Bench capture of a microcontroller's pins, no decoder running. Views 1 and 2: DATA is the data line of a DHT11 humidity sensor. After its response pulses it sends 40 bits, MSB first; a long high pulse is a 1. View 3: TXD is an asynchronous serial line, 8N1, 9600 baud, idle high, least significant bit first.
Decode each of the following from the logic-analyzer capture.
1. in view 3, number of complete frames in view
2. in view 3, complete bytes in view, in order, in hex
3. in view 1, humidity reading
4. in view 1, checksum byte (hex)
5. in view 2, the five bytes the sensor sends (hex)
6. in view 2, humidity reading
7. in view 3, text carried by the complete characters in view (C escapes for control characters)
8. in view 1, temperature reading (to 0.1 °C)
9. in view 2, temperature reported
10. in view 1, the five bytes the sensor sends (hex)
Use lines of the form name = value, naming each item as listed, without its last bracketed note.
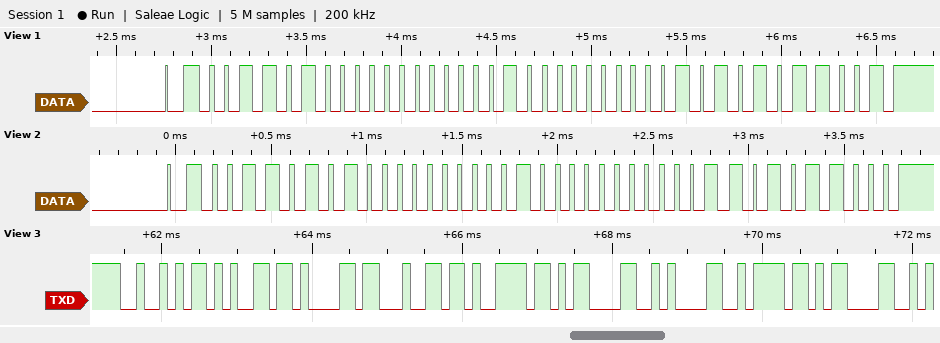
in view 3, number of complete frames in view = 9
in view 3, complete bytes in view, in order, in hex = 0x52 0x65 0x61 0x64 0x79 0x0D 0x0A 0x7A 0x0D
in view 1, humidity reading = 52 %
in view 1, checksum byte = 0x59
in view 2, the five bytes the sensor sends = 35 00 20 03 58
in view 2, humidity reading = 53 %
in view 3, text carried by the complete characters in view = "Ready\r\nz\r"
in view 1, temperature reading = 32.5 °C
in view 2, temperature reported = 32.3 °C
in view 1, the five bytes the sensor sends = 34 00 20 05 59
